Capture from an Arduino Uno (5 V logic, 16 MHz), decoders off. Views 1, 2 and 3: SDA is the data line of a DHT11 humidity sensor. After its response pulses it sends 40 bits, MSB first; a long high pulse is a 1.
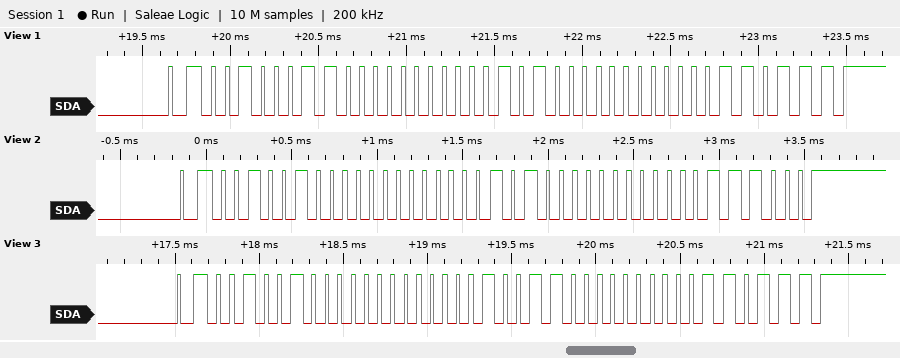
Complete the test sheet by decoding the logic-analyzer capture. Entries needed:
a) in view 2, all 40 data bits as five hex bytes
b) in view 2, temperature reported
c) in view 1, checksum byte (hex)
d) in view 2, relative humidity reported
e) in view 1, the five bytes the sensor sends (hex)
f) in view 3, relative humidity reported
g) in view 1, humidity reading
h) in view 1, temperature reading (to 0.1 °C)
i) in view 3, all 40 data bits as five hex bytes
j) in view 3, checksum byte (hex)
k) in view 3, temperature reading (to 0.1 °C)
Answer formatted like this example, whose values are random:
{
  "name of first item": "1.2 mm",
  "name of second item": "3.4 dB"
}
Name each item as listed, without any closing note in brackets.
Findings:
{
  "in view 2, all 40 data bits as five hex bytes": "24 00 14 00 38",
  "in view 2, temperature reported": "20.0 °C",
  "in view 1, checksum byte": "0x37",
  "in view 2, relative humidity reported": "36 %",
  "in view 1, the five bytes the sensor sends": "23 00 14 00 37",
  "in view 3, relative humidity reported": "36 %",
  "in view 1, humidity reading": "35 %",
  "in view 1, temperature reading": "20.0 °C",
  "in view 3, all 40 data bits as five hex bytes": "24 00 13 00 37",
  "in view 3, checksum byte": "0x37",
  "in view 3, temperature reading": "19.0 °C"
}
